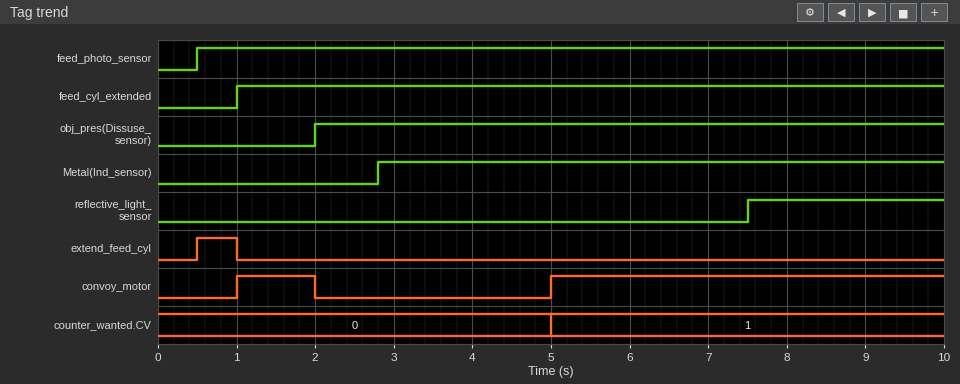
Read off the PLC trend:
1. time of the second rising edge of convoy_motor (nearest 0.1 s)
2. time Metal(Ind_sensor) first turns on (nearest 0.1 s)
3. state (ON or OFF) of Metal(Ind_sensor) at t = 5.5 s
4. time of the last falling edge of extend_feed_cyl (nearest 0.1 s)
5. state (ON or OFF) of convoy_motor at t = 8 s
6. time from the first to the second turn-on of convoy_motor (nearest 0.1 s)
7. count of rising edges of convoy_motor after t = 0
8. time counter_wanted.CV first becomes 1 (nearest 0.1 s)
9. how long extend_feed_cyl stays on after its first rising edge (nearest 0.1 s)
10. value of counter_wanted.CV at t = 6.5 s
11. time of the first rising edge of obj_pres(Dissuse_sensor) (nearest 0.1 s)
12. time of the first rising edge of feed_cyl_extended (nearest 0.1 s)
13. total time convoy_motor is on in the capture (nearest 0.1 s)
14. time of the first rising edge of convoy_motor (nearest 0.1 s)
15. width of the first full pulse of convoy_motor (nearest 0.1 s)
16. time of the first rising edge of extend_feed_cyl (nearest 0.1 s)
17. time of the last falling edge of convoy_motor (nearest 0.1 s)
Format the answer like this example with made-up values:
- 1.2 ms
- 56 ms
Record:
- 5.0 s
- 2.8 s
- ON
- 1.0 s
- ON
- 4.0 s
- 2
- 5.0 s
- 0.5 s
- 1
- 2.0 s
- 1.0 s
- 6.0 s
- 1.0 s
- 1.0 s
- 0.5 s
- 2.0 s
